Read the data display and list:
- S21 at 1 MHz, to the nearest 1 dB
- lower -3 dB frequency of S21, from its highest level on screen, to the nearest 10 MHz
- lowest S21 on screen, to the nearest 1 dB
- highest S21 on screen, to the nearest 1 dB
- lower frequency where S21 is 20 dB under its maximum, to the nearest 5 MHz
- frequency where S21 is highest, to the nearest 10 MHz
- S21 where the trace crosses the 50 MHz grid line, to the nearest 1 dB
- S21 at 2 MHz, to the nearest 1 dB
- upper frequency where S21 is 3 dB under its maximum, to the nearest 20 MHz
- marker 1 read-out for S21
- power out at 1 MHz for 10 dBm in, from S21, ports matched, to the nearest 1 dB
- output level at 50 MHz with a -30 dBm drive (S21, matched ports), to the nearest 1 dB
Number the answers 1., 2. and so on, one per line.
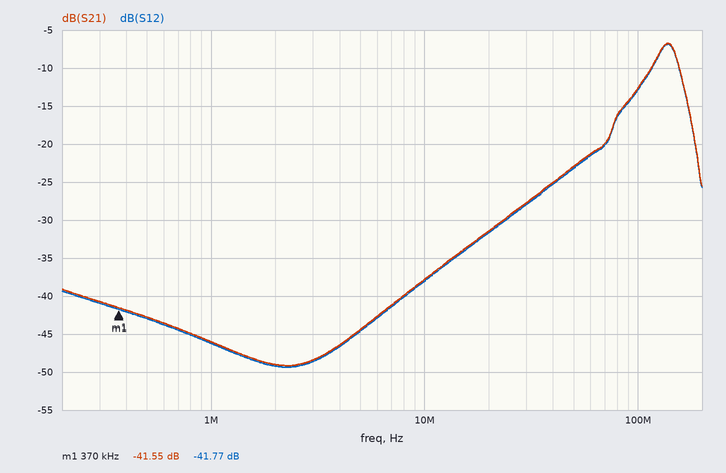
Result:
1. -46 dB
2. 120 MHz
3. -49 dB
4. -7 dB
5. 35 MHz
6. 140 MHz
7. -23 dB
8. -49 dB
9. 160 MHz
10. -41.55 dB
11. -36 dBm
12. -53 dBm
